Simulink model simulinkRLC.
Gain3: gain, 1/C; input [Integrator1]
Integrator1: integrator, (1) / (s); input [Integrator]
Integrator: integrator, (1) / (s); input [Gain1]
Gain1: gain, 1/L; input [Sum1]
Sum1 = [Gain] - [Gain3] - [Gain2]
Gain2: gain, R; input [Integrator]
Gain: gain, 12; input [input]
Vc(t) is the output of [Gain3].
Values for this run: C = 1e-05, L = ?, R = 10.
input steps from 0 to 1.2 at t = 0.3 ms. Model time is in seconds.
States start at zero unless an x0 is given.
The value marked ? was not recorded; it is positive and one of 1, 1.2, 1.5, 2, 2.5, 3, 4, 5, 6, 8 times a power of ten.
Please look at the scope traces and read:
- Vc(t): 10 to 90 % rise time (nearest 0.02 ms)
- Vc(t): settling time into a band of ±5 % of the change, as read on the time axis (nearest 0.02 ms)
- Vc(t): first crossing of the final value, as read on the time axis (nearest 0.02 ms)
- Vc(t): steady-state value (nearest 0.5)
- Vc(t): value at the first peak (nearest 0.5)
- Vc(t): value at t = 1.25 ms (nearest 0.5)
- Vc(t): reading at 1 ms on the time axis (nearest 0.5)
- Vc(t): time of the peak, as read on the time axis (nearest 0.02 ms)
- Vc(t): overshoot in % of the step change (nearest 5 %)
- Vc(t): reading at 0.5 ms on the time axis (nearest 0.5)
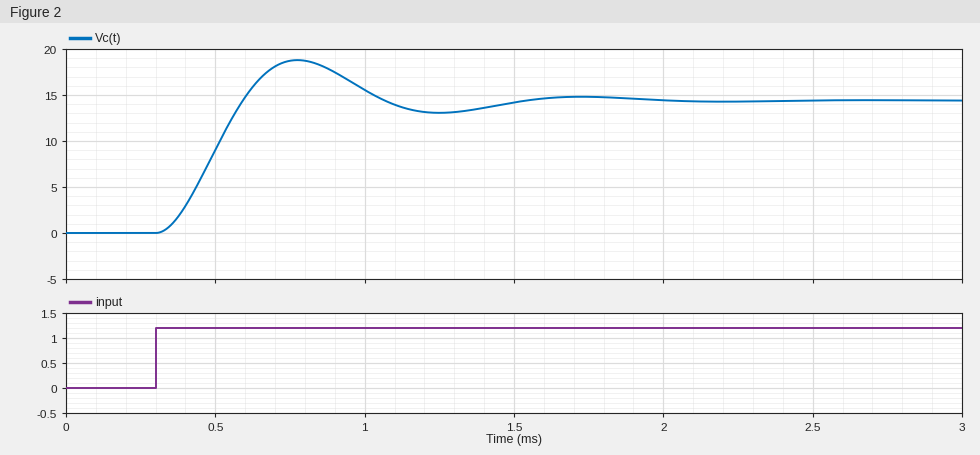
0.20 ms
1.42 ms
0.60 ms
14.5
19.0
13.0
15.5
0.78 ms
30 %
9.0
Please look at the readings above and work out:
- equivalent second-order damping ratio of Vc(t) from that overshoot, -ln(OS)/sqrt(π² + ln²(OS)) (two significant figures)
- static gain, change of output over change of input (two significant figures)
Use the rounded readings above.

0.36
12
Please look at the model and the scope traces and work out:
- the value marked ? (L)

0.002
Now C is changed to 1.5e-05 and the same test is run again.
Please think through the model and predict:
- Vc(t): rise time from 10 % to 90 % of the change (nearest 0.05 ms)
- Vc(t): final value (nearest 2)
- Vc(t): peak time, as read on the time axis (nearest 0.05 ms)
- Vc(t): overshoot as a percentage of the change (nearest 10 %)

0.25 ms
14
0.90 ms
20 %
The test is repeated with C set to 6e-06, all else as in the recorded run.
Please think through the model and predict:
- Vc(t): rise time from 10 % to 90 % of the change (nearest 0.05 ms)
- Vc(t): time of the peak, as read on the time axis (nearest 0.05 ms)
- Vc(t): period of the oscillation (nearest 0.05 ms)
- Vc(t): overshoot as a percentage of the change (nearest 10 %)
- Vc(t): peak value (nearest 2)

0.15 ms
0.65 ms
0.70 ms
40 %
20
